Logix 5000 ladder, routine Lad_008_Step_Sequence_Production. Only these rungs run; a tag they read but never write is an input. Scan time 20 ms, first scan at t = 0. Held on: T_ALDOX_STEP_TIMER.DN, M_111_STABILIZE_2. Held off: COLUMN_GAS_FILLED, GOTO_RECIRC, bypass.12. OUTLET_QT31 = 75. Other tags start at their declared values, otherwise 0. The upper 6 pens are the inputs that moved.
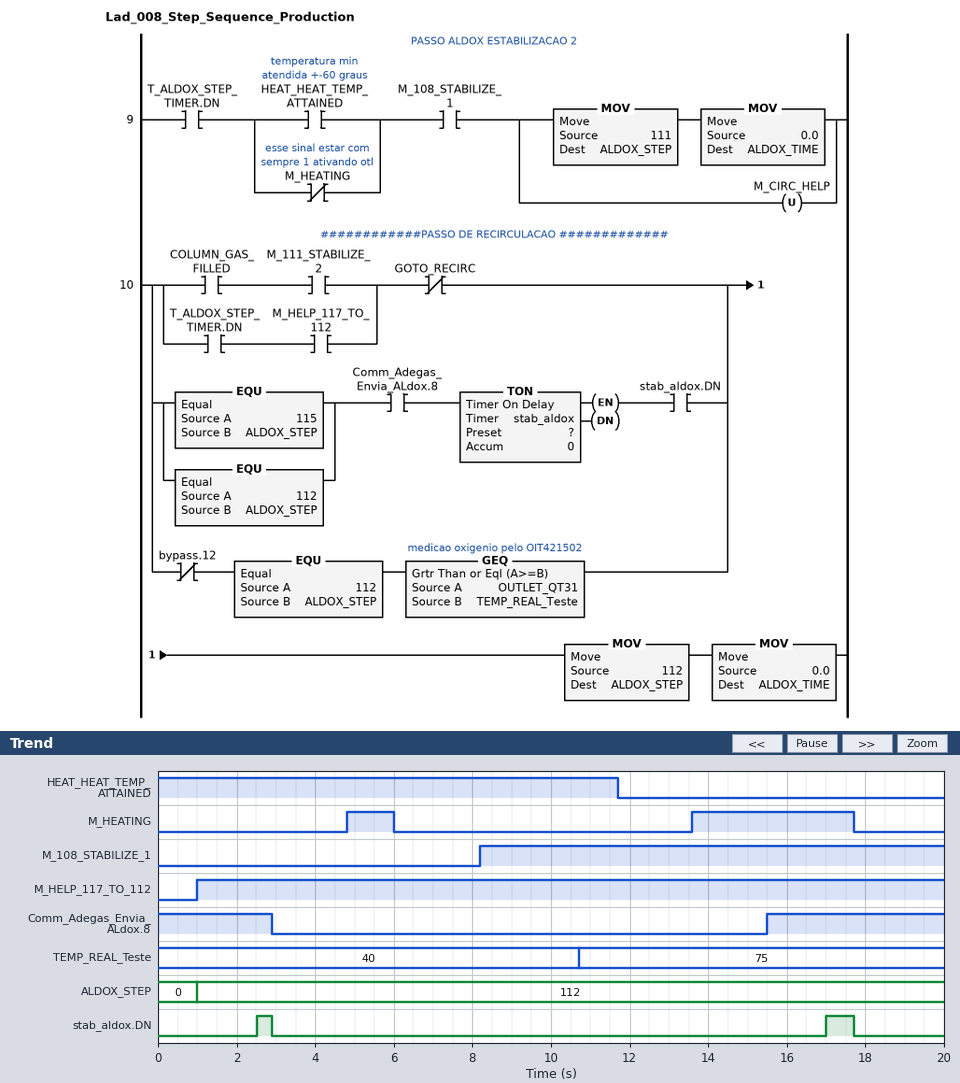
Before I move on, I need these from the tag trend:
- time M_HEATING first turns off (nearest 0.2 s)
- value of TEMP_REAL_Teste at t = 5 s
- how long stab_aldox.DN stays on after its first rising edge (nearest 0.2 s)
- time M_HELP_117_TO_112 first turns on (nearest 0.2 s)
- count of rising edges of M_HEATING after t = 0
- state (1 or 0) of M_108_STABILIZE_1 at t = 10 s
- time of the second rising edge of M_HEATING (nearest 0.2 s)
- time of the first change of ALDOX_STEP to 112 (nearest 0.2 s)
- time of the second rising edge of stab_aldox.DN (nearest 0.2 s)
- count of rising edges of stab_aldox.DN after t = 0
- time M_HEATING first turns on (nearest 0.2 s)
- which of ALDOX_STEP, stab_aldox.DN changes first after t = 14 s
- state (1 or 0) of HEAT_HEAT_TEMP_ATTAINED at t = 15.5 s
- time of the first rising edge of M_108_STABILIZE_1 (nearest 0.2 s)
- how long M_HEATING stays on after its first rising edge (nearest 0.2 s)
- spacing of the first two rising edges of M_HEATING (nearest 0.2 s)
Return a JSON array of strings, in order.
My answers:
["6.0 s", "40", "0.4 s", "1.0 s", "2", "1", "13.6 s", "1.0 s", "17.0 s", "2", "4.8 s", "stab_aldox.DN", "0", "8.2 s", "1.2 s", "8.8 s"]
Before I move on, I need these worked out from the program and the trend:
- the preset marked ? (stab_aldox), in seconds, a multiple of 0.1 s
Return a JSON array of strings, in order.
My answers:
["1.5 s"]
